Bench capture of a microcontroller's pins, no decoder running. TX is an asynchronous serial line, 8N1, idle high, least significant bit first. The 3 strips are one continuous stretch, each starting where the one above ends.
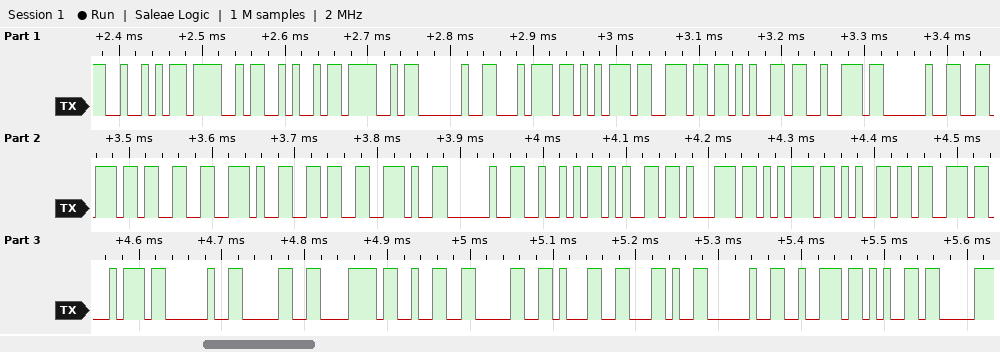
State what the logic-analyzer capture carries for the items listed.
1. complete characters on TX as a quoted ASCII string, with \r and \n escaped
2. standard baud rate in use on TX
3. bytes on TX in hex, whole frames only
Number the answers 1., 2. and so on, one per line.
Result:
1. "ROJO tuner v3.6. Request 0x201, re"
2. 115200 baud
3. 0x52 0x4F 0x4A 0x4F 0x20 0x74 0x75 0x6E 0x65 0x72 0x20 0x76 0x33 0x2E 0x36 0x2E 0x20 0x52 0x65 0x71 0x75 0x65 0x73 0x74 0x20 0x30 0x78 0x32 0x30 0x31 0x2C 0x20 0x72 0x65
